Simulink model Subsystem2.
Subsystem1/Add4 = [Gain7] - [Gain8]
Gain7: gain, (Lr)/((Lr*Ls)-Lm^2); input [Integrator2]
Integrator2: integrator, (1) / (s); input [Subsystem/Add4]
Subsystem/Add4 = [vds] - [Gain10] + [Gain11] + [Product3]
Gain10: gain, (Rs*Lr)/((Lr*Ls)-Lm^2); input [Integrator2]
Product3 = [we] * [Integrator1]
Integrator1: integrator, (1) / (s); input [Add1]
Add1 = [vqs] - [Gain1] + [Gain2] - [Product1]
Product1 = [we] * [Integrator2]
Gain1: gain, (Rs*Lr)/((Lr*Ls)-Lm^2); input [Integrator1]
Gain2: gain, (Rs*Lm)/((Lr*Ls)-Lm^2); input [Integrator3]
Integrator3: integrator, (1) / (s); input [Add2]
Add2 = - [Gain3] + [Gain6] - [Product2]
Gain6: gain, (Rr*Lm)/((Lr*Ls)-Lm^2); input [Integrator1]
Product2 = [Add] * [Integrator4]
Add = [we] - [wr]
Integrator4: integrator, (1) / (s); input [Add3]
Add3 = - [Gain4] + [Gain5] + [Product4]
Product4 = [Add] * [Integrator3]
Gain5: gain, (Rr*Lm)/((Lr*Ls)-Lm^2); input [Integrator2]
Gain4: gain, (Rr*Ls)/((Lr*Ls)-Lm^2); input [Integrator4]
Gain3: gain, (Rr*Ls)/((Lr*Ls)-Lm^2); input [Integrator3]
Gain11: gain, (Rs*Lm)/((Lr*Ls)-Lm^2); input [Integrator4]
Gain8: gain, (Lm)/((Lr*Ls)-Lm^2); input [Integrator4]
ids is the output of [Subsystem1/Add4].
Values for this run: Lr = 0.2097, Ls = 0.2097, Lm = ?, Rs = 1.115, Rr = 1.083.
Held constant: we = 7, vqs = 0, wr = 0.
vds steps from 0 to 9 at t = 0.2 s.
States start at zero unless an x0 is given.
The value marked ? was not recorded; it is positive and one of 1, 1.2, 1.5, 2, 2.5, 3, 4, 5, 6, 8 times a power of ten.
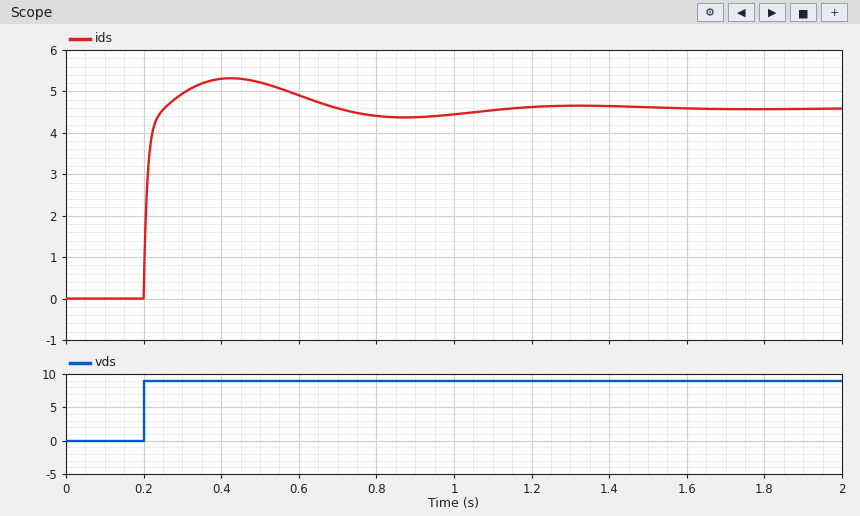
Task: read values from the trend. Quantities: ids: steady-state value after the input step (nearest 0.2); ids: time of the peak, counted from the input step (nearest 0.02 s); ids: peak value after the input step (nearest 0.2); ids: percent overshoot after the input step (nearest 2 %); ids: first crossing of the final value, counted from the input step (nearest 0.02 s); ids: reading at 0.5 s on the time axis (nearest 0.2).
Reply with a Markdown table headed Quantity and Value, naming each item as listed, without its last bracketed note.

| Quantity | Value |
|---|---|
| ids: steady-state value after the input step | 4.6 |
| ids: time of the peak, counted from the input step | 0.22 s |
| ids: peak value after the input step | 5.4 |
| ids: percent overshoot after the input step | 16 % |
| ids: first crossing of the final value, counted from the input step | 0.06 s |
| ids: reading at 0.5 s on the time axis | 5.2 |
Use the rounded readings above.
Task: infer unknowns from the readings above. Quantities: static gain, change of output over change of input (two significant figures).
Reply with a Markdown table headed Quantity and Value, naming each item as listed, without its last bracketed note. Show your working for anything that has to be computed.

| Quantity | Value |
|---|---|
| static gain, change of output over change of input | (4.6 - 0) / (9 - 0) = 0.51 |
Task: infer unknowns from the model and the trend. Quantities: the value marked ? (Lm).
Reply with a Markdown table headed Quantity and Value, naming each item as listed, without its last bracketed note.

| Quantity | Value |
|---|---|
| the value marked ? | 0.2 |
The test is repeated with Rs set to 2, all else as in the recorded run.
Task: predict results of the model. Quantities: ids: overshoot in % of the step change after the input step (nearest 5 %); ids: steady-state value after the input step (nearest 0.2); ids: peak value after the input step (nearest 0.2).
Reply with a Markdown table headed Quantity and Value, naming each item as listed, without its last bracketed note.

| Quantity | Value |
|---|---|
| ids: overshoot in % of the step change after the input step | 10 % |
| ids: steady-state value after the input step | 3.2 |
| ids: peak value after the input step | 3.6 |
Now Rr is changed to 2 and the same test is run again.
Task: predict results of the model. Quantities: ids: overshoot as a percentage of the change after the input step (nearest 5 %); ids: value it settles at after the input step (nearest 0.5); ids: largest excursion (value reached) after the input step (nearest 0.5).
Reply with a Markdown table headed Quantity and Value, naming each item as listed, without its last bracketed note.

| Quantity | Value |
|---|---|
| ids: overshoot as a percentage of the change after the input step | 25 % |
| ids: value it settles at after the input step | 4.0 |
| ids: largest excursion (value reached) after the input step | 5.0 |
